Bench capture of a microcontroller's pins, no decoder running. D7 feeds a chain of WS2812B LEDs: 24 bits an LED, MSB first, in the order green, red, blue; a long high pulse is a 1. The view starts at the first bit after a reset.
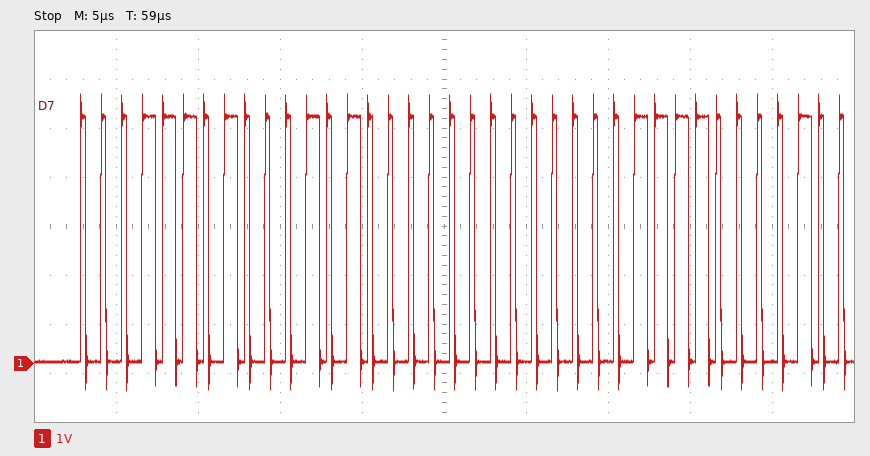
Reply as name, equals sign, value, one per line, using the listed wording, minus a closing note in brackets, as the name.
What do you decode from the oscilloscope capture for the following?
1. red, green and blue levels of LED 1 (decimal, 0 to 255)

red, green and blue levels of LED 1 = 20, 29, 0
